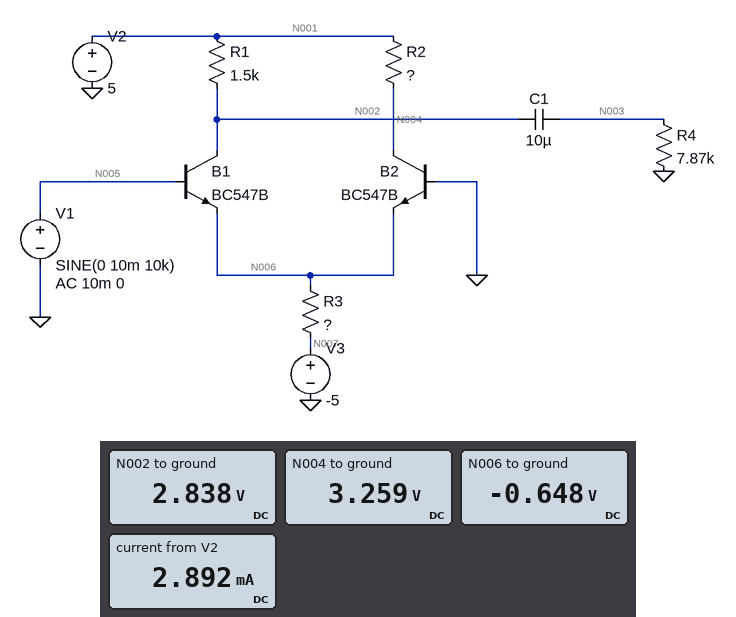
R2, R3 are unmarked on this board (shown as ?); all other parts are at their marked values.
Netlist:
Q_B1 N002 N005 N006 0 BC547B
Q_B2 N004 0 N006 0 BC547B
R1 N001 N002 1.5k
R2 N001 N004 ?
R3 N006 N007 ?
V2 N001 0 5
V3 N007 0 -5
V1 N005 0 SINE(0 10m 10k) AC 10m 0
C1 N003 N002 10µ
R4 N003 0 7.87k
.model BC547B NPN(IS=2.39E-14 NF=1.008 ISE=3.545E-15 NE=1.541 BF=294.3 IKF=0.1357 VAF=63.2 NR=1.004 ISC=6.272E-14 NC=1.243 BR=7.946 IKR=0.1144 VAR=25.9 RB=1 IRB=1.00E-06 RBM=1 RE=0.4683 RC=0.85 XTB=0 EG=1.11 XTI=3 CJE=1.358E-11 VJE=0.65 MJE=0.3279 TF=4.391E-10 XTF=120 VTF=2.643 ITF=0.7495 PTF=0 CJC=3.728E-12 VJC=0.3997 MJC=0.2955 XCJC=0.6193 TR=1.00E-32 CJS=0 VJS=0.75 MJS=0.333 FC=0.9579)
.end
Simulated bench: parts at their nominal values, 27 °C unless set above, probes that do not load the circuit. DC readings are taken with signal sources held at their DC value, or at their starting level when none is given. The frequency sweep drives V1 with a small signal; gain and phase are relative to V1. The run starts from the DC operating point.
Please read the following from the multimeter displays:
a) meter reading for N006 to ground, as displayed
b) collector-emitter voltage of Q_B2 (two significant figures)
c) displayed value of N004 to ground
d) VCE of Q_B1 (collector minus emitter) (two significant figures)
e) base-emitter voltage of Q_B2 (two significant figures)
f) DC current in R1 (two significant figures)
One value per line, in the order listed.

-0.648 V
3.9 V
3.259 V
3.5 V
650 mV
1.4 mA
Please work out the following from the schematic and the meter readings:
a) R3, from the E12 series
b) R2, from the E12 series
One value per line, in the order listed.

1.5 kΩ
1.2 kΩ
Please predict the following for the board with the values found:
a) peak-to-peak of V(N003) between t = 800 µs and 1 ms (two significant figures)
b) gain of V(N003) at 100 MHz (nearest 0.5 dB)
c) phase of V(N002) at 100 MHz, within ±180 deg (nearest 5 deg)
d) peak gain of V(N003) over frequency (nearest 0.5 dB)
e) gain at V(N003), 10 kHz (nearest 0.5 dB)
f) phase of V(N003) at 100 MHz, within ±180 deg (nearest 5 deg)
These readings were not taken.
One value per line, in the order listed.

650 mV
25.0 dB
115 deg
30.5 dB
30.5 dB
115 deg
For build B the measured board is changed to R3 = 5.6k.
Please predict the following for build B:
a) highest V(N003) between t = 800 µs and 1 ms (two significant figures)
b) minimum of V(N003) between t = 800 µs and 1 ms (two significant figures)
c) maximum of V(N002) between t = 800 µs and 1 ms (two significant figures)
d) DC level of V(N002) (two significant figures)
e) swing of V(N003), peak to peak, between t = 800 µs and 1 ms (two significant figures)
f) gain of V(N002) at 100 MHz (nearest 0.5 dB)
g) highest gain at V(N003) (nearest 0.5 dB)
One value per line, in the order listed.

92 mV
-92 mV
4.5 V
4.4 V
180 mV
14.5 dB
19.5 dB
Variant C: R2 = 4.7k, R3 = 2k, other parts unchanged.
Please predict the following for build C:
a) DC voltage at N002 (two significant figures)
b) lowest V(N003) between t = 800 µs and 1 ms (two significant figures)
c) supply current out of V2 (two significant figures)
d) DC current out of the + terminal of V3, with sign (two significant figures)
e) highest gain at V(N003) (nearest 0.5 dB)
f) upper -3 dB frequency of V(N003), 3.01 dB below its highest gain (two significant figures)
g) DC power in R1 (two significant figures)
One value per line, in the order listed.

3.3 V
-240 mV
2.2 mA
-2.2 mA
28.0 dB
69 MHz
1.9 mW
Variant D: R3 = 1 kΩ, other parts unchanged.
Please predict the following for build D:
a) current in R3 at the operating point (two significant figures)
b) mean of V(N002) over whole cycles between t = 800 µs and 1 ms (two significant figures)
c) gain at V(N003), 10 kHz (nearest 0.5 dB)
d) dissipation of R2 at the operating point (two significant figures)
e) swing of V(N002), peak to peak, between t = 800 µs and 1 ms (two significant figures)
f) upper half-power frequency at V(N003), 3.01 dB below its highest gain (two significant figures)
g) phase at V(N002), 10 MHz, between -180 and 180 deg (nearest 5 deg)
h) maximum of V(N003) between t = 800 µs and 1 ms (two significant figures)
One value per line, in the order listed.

4.3 mA
1.8 V
33.5 dB
5.7 mW
950 mV
55 MHz
170 deg
470 mV
